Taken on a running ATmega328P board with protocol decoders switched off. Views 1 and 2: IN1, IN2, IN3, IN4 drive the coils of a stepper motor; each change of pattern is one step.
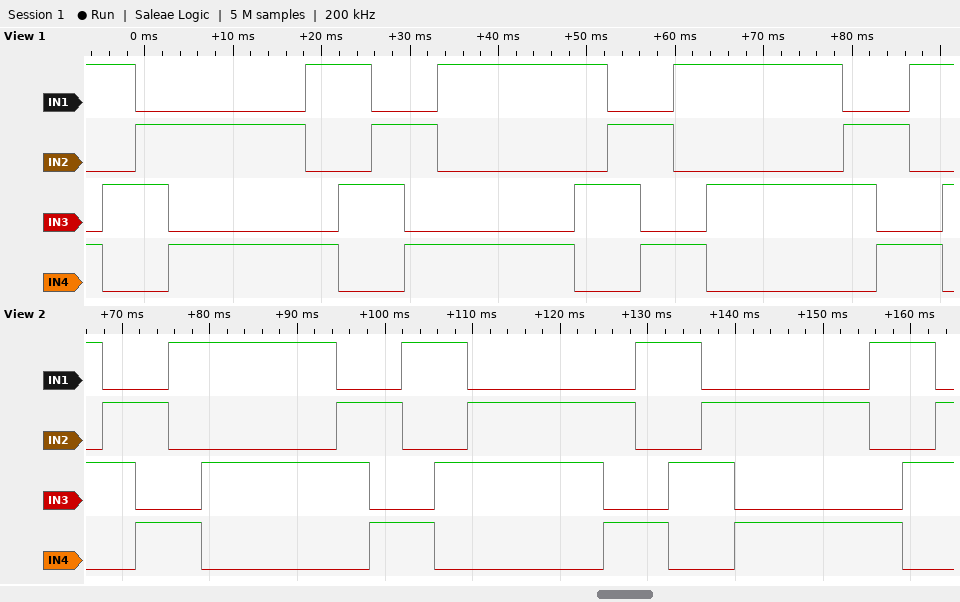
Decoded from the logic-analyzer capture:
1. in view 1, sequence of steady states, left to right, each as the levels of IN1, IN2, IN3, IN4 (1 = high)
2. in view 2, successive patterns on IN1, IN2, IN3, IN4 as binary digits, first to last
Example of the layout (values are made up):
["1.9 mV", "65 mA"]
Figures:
["1001 1010 0110 0101 1001 1010 0110 0101 1001 1010 0110 0101 1001 1010 0110 0101 1001 1010", "1010 0110 0101 1001 1010 0110 0101 1001 1010 0110 0101 1001 1010 0110 0101 1001 1010 0110"]
